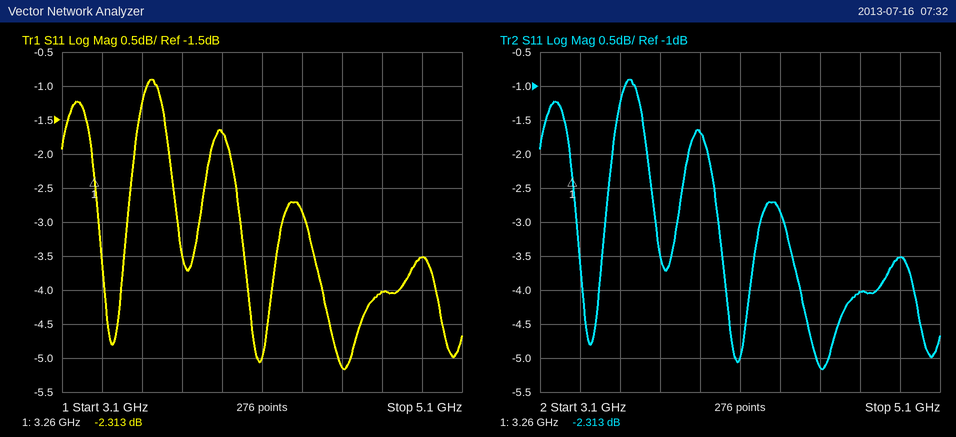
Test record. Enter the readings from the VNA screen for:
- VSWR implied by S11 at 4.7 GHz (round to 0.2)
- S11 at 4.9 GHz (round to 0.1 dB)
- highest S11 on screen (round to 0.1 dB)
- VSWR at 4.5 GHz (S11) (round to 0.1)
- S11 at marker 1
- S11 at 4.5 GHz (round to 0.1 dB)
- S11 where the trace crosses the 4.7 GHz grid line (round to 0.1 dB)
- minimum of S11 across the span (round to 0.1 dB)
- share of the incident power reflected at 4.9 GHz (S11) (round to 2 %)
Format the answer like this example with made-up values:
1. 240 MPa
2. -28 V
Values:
1. 4.4
2. -3.5 dB
3. -0.9 dB
4. 3.5
5. -2.313 dB
6. -5.1 dB
7. -4.0 dB
8. -5.2 dB
9. 44 %
